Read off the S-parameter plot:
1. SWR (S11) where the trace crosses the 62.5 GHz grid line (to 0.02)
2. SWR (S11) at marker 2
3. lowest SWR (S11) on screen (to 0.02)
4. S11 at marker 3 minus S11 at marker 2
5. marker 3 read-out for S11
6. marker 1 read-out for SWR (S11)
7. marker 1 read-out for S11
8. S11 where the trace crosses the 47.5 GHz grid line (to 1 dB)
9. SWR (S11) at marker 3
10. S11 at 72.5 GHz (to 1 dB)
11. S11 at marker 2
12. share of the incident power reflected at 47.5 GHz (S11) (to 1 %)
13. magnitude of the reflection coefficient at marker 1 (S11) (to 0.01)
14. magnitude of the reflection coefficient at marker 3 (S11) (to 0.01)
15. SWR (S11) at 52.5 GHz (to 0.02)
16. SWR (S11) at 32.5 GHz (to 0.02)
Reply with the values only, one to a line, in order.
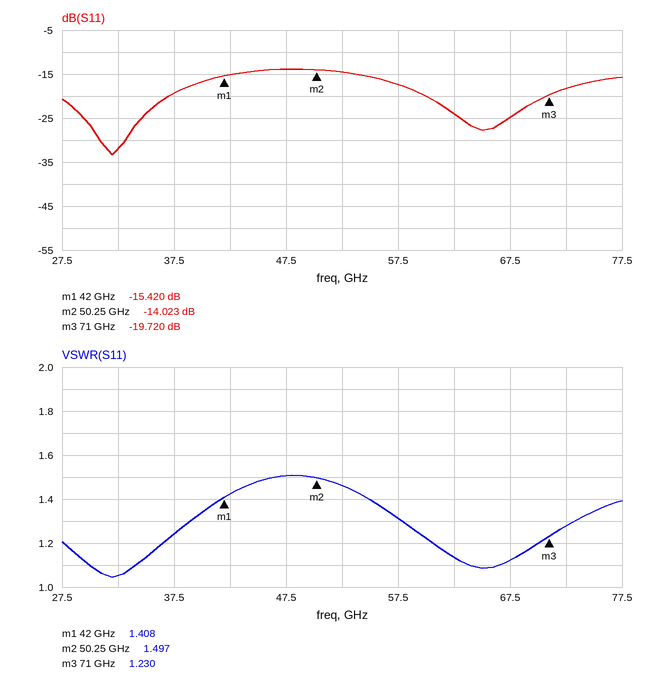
1.14
1.497
1.04
-5.697 dB
-19.720 dB
1.408
-15.420 dB
-14 dB
1.230
-18 dB
-14.023 dB
4 %
0.17
0.10
1.46
1.06
